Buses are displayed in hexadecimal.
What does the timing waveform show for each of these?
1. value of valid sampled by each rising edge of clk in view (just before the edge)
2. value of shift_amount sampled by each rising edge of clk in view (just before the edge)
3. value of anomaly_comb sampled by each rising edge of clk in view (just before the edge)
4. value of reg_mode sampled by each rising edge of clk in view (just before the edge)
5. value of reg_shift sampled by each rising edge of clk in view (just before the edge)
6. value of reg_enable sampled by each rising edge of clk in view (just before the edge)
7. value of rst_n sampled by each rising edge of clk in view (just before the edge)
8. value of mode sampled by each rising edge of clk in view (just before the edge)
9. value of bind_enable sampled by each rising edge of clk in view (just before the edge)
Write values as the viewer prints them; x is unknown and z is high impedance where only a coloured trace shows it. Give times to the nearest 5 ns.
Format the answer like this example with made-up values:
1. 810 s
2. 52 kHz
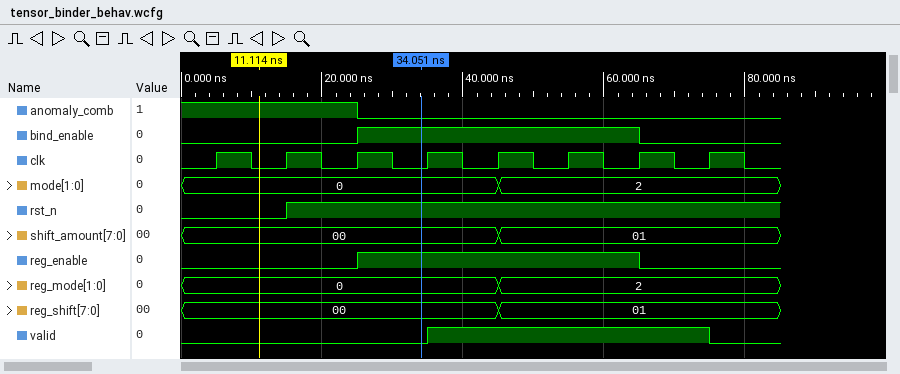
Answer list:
1. 0 0 0 0 1 1 1 1
2. 00, 00, 00, 00, 00, 01, 01, 01
3. 1 1 1 0 0 0 0 0
4. 0, 0, 0, 0, 0, 2, 2, 2
5. 00, 00, 00, 00, 00, 01, 01, 01
6. 0 0 0 1 1 1 1 0
7. 0 0 1 1 1 1 1 1
8. 0, 0, 0, 0, 0, 2, 2, 2
9. 0 0 0 1 1 1 1 0
